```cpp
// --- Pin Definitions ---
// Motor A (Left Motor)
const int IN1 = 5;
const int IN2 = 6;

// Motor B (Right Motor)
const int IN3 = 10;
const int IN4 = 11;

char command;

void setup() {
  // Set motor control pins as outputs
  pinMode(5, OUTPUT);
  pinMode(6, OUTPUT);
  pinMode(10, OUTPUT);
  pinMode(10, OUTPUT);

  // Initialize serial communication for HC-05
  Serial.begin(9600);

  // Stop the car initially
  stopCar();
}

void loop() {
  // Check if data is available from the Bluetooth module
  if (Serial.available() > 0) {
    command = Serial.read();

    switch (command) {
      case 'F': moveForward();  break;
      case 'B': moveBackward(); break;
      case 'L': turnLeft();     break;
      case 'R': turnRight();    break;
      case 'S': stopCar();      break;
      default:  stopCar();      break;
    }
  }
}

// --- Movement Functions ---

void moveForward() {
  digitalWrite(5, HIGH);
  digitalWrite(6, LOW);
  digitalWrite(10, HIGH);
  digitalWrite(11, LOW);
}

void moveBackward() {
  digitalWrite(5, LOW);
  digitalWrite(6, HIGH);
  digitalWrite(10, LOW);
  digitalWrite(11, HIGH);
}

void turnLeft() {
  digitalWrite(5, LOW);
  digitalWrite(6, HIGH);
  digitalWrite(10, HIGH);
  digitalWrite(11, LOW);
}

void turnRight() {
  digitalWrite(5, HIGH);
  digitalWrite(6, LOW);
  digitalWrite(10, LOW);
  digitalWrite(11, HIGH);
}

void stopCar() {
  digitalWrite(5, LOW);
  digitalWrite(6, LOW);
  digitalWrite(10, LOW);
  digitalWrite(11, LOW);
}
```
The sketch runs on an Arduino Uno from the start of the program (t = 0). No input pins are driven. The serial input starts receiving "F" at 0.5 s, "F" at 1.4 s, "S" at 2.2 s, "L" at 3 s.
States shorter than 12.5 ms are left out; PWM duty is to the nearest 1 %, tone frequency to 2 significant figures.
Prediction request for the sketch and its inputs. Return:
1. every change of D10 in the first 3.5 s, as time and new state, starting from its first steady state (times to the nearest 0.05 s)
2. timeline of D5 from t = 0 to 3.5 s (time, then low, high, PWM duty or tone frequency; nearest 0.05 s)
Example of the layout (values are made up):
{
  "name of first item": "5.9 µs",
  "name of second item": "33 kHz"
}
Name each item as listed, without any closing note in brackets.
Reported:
{
  "every change of D10 in the first 3.5 s, as time and new state, starting from its first steady state": "0 s low; 0.5 s high; 2.2 s low; 3 s high",
  "timeline of D5 from t = 0 to 3.5 s": "0 s low; 0.5 s high; 2.2 s low"
}
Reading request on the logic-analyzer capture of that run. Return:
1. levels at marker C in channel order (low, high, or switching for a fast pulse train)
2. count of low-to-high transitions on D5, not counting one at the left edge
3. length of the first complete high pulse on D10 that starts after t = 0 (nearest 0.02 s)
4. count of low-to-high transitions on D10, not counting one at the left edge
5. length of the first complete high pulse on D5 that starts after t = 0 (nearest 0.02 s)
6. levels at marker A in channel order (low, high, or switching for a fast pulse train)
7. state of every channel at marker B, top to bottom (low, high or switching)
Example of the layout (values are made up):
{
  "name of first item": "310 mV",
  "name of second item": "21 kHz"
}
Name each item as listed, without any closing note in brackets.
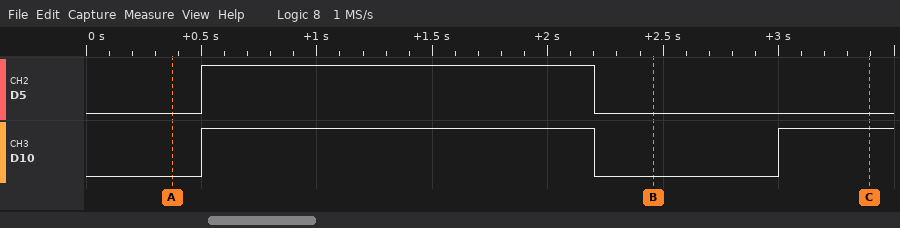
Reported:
{
  "levels at marker C in channel order": "D5 low, D10 high",
  "count of low-to-high transitions on D5, not counting one at the left edge": "1",
  "length of the first complete high pulse on D10 that starts after t = 0": "1.70 s",
  "count of low-to-high transitions on D10, not counting one at the left edge": "2",
  "length of the first complete high pulse on D5 that starts after t = 0": "1.70 s",
  "levels at marker A in channel order": "D5 low, D10 low",
  "state of every channel at marker B, top to bottom": "D5 low, D10 low"
}
